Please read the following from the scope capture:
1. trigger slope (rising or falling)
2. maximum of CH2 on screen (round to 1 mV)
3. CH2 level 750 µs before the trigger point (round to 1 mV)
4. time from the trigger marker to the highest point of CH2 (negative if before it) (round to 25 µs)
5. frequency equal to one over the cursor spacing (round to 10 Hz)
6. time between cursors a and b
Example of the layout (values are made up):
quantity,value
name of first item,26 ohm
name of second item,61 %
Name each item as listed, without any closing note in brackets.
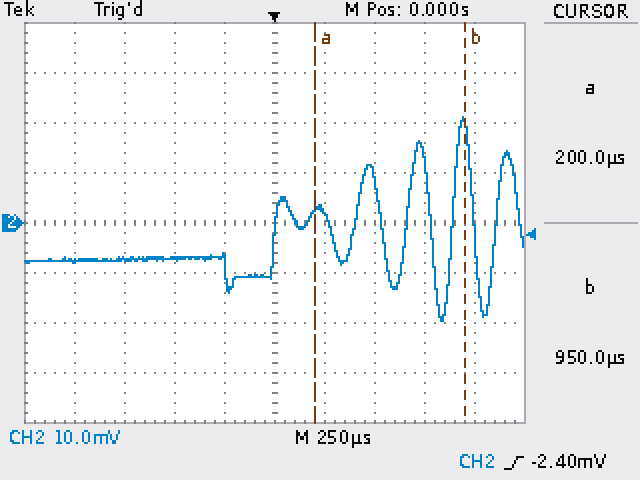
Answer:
quantity,value
trigger slope,rising
maximum of CH2 on screen,21 mV
CH2 level 750 µs before the trigger point,-7 mV
time from the trigger marker to the highest point of CH2 (negative if before it),+950 µs
frequency equal to one over the cursor spacing,1.33 kHz
time between cursors a and b,750 µs
